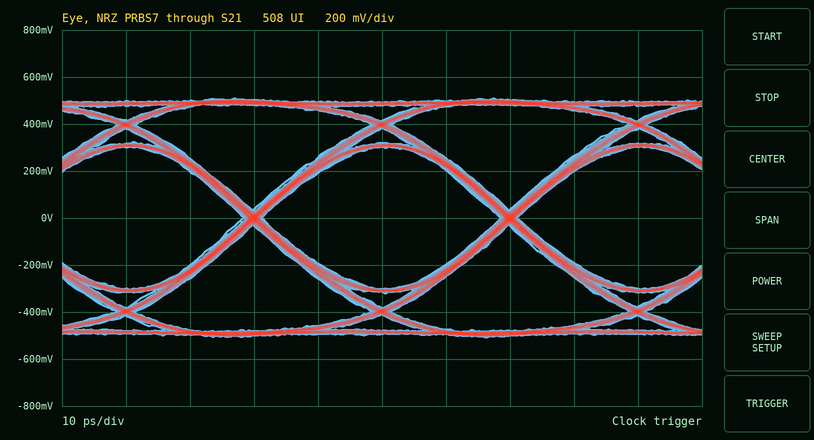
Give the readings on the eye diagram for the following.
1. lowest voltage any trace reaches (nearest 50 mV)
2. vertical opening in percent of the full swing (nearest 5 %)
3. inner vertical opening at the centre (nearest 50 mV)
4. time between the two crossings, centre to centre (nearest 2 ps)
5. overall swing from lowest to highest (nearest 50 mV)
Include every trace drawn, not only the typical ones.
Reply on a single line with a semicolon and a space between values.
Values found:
-500 mV; 60 %; 600 mV; 40 ps; 1.00 V
